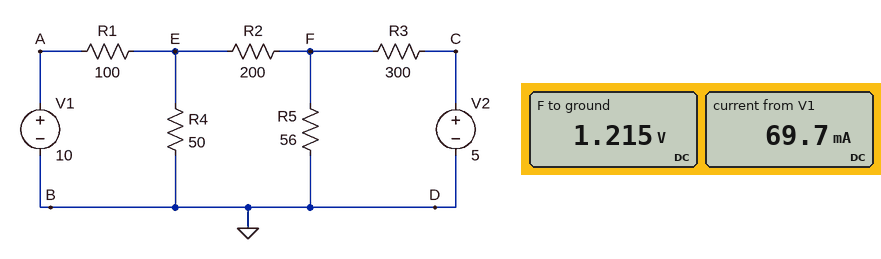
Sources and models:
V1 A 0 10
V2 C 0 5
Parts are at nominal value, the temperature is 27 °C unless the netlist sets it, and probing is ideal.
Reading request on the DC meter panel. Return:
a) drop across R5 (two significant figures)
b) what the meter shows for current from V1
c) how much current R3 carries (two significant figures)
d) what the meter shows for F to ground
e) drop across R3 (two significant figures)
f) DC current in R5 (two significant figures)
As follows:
1.2 V
69.7 mA
13 mA
1.215 V
3.8 V
22 mA
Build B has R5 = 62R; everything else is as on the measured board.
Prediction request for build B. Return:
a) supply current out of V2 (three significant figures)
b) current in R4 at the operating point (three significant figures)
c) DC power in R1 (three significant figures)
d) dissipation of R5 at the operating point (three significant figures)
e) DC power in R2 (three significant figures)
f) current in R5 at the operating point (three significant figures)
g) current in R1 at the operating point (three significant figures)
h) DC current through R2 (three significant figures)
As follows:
12.3 mA
60.9 mA
484 mW
27.4 mW
15.1 mW
21.0 mA
69.6 mA
8.70 mA
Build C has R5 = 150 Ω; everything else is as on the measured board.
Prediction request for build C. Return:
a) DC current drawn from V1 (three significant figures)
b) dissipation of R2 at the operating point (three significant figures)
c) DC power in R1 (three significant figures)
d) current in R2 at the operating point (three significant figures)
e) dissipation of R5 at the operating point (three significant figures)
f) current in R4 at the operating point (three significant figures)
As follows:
68.3 mA
5.00 mW
467 mW
5.00 mA
31.3 mW
63.3 mA
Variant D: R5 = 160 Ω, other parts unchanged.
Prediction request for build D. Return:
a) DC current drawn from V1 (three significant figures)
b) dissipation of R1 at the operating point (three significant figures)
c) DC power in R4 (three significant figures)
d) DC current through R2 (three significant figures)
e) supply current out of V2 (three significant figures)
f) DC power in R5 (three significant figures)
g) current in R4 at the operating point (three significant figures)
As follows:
68.2 mA
466 mW
202 mW
4.72 mA
9.23 mA
31.1 mW
63.5 mA
